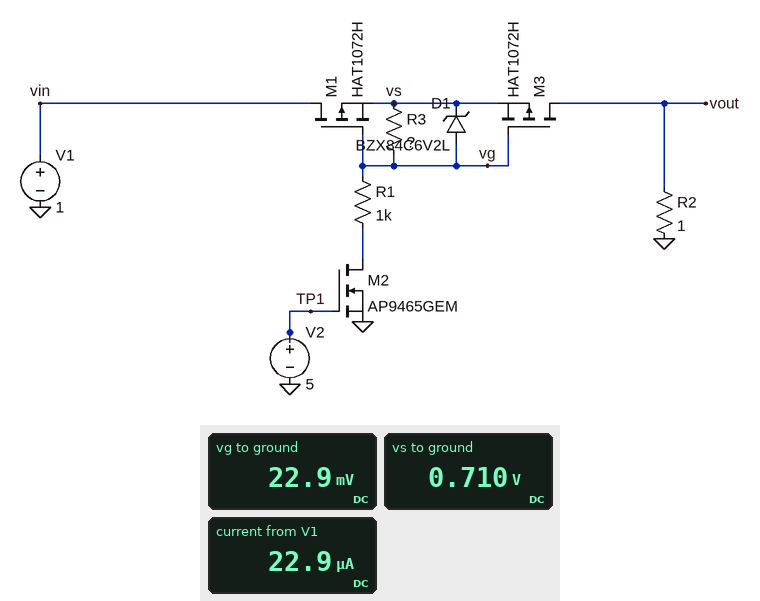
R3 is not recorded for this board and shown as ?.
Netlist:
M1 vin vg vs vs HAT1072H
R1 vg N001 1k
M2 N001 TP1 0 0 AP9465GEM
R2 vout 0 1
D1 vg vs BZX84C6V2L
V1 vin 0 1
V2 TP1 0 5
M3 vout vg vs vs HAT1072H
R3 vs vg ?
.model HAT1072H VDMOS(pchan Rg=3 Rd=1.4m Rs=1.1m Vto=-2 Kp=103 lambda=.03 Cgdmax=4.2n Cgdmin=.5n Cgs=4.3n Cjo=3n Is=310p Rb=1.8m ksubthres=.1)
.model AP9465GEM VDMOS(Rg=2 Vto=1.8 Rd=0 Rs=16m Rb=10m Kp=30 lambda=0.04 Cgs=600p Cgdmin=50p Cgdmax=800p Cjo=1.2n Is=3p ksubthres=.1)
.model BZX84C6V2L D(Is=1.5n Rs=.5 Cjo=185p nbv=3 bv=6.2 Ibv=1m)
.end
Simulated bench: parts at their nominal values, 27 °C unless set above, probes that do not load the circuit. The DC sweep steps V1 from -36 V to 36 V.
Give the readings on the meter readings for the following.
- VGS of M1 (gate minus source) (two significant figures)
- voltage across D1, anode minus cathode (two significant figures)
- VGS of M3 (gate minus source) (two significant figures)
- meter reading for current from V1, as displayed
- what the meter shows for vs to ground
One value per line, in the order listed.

-690 mV
-690 mV
-690 mV
22.9 µA
0.710 V
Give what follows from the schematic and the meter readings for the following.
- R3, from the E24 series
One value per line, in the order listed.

30 kΩ
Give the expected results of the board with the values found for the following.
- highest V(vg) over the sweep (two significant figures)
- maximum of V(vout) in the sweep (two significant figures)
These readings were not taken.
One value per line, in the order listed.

29 V
36 V
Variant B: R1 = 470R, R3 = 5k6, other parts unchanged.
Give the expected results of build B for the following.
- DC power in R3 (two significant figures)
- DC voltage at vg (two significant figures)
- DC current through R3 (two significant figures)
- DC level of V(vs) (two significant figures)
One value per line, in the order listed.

68 µW
52 mV
110 µA
670 mV
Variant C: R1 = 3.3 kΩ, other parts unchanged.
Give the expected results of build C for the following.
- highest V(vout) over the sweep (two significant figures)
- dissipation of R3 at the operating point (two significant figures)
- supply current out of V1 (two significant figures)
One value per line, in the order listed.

36 V
14 µW
21 µA
